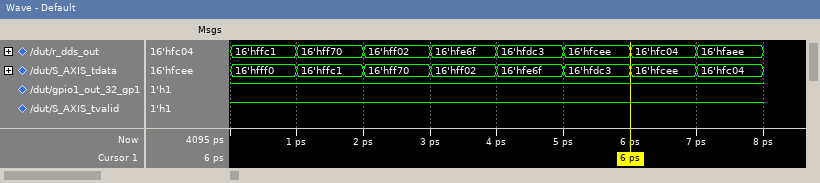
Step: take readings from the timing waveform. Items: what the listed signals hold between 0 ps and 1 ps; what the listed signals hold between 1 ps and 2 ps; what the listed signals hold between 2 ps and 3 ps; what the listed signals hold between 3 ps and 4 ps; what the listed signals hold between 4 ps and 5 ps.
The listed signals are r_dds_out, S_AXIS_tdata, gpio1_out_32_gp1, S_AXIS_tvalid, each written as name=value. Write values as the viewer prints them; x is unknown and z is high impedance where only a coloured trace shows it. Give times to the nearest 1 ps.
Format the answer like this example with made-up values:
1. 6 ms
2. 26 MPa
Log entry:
1. r_dds_out=16'hffc1, S_AXIS_tdata=16'hfff0, gpio1_out_32_gp1=1, S_AXIS_tvalid=1
2. r_dds_out=16'hff70, S_AXIS_tdata=16'hffc1, gpio1_out_32_gp1=1, S_AXIS_tvalid=1
3. r_dds_out=16'hff02, S_AXIS_tdata=16'hff70, gpio1_out_32_gp1=1, S_AXIS_tvalid=1
4. r_dds_out=16'hfe6f, S_AXIS_tdata=16'hff02, gpio1_out_32_gp1=1, S_AXIS_tvalid=1
5. r_dds_out=16'hfdc3, S_AXIS_tdata=16'hfe6f, gpio1_out_32_gp1=1, S_AXIS_tvalid=1
